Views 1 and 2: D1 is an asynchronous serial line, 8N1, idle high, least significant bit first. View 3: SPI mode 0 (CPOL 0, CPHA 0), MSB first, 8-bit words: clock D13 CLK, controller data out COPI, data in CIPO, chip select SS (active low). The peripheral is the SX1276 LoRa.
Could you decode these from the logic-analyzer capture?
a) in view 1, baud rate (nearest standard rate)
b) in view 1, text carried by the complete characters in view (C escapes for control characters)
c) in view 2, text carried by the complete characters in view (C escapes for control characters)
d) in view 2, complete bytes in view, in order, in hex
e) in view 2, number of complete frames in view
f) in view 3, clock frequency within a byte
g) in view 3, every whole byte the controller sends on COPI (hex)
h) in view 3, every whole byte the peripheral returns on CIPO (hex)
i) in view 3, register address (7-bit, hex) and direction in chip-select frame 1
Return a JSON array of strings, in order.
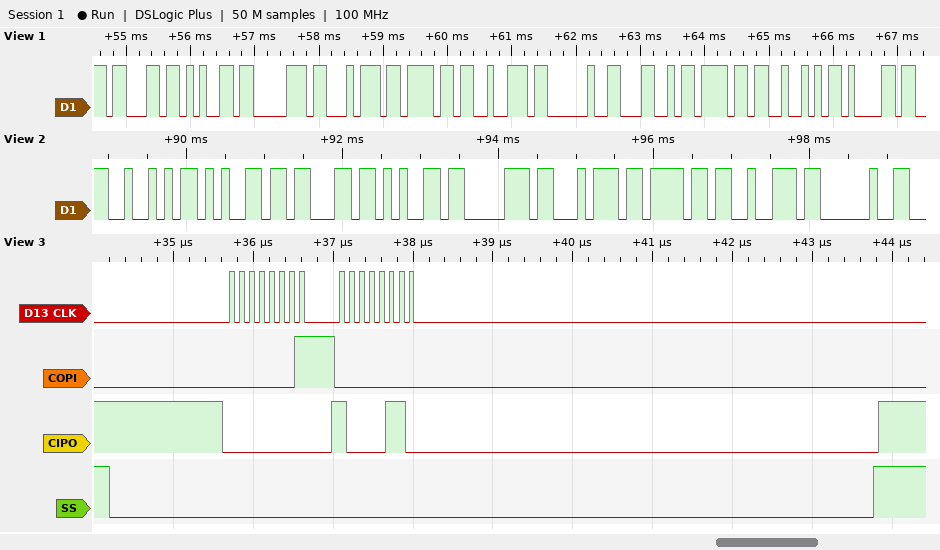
["9600 baud", "\"ceptor LoRa\"", "\"Receptor \"", "0x52 0x65 0x63 0x65 0x70 0x74 0x6F 0x72 0x20", "9", "8 MHz", "01 00", "00 86", "0x01 read"]
